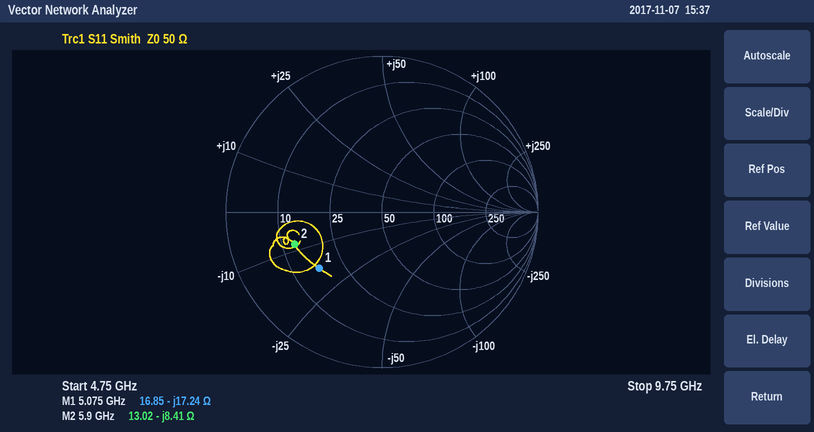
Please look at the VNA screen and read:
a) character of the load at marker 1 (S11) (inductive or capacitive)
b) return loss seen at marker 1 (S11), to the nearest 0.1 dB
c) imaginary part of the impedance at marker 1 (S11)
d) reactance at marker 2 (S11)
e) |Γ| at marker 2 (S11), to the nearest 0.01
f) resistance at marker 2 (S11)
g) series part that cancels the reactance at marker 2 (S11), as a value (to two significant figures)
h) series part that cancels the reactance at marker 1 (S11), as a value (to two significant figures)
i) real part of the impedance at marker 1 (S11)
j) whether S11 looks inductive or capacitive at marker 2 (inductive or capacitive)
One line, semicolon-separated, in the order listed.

capacitive; 5.3 dB; -17.24 Ω; -8.41 Ω; 0.60; 13.02 Ω; 230 pH; 540 pH; 16.85 Ω; capacitive
